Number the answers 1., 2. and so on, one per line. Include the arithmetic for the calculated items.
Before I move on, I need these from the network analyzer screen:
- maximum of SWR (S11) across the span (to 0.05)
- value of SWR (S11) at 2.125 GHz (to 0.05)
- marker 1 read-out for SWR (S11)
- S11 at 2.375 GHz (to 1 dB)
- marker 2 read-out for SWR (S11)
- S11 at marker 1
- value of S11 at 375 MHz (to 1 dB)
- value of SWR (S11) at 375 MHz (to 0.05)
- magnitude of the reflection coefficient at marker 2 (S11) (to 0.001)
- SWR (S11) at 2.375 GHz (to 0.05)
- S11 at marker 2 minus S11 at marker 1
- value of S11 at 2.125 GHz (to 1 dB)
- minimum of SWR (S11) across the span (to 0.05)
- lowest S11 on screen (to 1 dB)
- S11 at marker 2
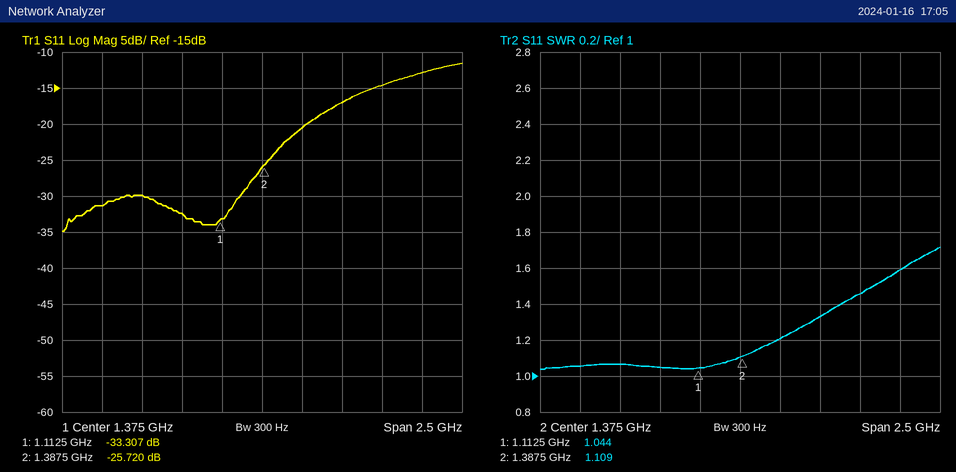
1. 1.70
2. 1.45
3. 1.044
4. -13 dB
5. 1.109
6. -33.307 dB
7. -31 dB
8. 1.05
9. 10^(-25.72/20) ≈ 0.052
10. 1.60
11. -25.72 − (-33.307) = 7.587 dB
12. -15 dB
13. 1.05
14. -35 dB
15. -25.720 dB
